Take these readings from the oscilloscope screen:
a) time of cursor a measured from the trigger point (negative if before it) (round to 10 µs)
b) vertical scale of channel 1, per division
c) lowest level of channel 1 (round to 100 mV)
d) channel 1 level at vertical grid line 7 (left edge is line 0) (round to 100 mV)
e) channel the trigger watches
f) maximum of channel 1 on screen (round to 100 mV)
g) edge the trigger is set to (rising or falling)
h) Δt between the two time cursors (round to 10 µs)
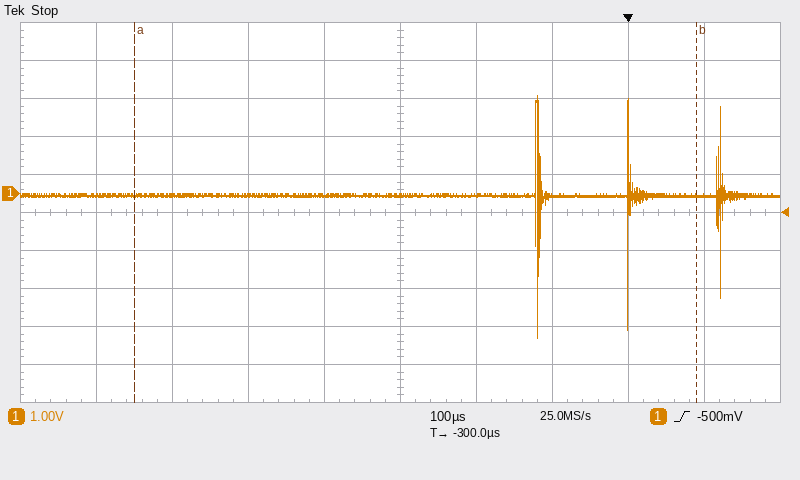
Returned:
-650 µs
1 V
-3.8 V
-100 mV
channel 1
2.6 V
rising
740 µs
